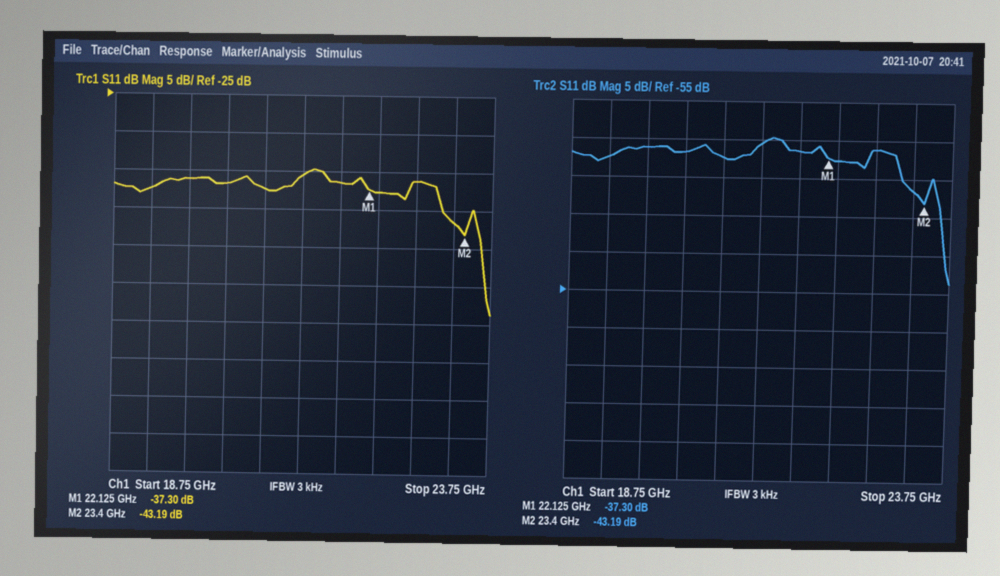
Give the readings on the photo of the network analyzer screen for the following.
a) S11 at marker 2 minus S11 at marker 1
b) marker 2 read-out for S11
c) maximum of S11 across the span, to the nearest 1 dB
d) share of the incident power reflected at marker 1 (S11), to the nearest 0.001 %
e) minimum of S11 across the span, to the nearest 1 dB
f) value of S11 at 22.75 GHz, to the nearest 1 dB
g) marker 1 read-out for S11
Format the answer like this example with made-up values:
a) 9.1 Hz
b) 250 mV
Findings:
a) -5.89 dB
b) -43.19 dB
c) -35 dB
d) 0.019 %
e) -54 dB
f) -36 dB
g) -37.30 dB
